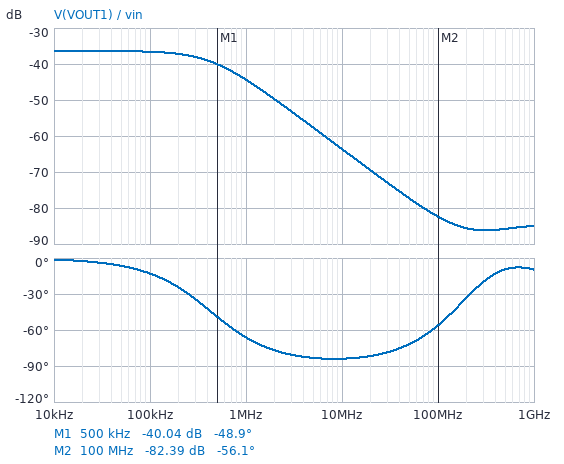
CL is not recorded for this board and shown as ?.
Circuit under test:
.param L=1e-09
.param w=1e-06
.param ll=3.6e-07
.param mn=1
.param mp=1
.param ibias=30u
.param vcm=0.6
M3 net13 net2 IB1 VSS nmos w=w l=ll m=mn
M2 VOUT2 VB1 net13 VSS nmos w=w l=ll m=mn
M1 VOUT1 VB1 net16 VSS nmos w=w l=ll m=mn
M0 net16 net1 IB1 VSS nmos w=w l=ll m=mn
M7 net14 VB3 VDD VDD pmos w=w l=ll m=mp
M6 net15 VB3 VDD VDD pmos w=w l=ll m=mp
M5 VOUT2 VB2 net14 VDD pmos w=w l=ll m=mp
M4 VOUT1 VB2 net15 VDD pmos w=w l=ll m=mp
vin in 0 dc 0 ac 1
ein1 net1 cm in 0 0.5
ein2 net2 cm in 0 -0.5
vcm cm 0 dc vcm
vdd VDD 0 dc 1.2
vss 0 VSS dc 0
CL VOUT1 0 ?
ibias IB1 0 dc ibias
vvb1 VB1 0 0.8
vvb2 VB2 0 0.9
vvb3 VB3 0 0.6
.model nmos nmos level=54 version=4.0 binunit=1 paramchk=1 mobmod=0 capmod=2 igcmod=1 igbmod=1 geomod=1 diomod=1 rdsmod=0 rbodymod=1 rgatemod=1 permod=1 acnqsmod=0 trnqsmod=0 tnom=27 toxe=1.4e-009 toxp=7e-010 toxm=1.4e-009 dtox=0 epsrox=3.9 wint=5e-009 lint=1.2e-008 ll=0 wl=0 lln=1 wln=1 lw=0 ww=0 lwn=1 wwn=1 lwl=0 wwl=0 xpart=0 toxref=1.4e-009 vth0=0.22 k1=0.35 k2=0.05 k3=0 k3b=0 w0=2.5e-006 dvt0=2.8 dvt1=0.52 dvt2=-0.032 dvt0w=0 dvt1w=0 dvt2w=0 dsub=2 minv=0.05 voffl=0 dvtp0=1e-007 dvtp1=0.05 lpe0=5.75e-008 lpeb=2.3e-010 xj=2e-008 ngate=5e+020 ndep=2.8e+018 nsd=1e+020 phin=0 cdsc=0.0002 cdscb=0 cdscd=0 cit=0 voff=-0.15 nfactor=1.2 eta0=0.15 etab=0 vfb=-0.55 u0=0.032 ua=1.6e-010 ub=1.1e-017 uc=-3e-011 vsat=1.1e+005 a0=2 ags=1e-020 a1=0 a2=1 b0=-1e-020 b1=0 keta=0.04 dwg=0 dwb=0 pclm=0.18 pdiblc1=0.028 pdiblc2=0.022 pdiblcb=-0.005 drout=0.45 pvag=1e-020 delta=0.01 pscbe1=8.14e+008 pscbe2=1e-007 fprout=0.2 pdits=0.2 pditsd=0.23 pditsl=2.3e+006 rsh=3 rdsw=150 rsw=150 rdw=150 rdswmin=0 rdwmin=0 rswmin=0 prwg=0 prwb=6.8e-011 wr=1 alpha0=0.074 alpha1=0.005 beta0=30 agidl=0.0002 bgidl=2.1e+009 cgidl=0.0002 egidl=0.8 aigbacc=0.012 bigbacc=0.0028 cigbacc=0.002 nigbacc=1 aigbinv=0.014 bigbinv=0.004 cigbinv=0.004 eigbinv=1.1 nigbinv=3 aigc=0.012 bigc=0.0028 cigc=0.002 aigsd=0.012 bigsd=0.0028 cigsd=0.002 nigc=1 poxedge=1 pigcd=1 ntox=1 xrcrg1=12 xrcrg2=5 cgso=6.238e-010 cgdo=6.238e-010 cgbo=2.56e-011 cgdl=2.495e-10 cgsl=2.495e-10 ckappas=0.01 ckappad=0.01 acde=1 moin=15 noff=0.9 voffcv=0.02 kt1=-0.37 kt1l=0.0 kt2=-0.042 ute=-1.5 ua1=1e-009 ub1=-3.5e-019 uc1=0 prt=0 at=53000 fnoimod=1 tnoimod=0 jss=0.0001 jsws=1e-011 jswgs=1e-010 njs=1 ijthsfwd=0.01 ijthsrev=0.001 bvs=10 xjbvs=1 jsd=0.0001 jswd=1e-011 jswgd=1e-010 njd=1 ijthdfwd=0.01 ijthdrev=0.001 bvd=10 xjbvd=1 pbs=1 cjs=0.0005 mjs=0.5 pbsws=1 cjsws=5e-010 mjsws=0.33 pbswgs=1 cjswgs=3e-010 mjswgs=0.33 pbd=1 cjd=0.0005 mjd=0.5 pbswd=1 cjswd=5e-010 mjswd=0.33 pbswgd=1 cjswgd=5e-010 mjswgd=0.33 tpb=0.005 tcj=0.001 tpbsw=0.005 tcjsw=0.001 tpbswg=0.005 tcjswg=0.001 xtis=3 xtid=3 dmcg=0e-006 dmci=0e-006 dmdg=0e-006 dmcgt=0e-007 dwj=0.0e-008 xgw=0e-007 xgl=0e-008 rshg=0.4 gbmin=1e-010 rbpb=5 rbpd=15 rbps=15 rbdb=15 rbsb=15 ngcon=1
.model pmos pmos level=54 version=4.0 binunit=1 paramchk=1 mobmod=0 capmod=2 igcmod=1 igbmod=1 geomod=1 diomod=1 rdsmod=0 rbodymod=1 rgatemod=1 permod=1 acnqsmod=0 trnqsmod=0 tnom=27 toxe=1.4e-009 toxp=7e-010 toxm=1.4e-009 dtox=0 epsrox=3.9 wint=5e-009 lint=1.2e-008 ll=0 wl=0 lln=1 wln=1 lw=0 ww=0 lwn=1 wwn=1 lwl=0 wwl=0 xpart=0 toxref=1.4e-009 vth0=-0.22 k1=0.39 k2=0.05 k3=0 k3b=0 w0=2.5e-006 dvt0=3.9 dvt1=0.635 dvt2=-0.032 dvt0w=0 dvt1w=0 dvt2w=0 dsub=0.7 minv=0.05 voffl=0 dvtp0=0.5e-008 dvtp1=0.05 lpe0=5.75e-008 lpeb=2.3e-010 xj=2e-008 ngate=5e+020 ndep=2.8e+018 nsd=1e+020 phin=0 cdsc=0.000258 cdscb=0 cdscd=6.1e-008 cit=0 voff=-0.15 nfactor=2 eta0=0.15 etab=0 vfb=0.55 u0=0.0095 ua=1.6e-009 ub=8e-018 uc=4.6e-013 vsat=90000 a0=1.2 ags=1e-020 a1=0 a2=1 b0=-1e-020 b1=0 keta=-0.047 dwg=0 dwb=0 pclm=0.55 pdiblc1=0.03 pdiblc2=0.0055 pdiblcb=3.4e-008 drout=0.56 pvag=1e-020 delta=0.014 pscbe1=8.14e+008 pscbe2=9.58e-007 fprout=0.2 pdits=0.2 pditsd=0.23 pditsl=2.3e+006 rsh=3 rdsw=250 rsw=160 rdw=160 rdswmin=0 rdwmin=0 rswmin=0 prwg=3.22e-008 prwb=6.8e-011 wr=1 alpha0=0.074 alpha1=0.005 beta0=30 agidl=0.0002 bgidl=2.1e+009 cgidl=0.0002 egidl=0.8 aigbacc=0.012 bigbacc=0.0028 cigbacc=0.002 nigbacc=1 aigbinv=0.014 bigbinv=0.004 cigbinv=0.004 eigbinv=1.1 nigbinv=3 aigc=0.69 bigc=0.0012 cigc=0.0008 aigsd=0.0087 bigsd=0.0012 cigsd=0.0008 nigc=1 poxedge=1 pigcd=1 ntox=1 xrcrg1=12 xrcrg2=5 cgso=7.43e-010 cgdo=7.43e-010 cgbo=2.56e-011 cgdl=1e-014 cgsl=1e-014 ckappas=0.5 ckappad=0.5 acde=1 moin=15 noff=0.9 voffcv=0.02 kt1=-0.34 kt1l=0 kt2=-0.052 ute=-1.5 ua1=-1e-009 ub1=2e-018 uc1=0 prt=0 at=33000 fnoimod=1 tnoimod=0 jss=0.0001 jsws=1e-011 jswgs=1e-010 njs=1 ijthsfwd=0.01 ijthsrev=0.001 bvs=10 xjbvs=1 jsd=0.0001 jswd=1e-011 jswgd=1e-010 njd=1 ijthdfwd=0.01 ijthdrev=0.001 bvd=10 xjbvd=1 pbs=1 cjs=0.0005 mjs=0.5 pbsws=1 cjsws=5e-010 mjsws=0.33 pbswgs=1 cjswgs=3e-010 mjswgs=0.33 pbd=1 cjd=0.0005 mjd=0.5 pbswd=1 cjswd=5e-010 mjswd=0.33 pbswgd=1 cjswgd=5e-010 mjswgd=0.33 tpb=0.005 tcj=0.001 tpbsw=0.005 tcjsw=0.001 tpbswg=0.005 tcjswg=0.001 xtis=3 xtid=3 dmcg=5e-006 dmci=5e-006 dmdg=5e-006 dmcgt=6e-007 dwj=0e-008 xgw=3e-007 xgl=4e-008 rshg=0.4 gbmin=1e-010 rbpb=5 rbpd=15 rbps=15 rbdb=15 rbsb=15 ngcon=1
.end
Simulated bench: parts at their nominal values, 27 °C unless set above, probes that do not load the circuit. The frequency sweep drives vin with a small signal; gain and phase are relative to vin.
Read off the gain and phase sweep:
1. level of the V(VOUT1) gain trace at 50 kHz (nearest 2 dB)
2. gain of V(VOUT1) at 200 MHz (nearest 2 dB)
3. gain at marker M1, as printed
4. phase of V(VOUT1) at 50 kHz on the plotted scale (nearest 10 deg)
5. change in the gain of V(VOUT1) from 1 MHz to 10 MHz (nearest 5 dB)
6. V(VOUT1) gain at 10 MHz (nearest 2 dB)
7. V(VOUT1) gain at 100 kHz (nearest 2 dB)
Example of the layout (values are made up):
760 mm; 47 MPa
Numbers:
-36 dB; -86 dB; -40.04 dB; -10 deg; -20 dB; -64 dB; -36 dB
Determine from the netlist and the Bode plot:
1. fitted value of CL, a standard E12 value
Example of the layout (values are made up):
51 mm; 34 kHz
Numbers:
33 pF
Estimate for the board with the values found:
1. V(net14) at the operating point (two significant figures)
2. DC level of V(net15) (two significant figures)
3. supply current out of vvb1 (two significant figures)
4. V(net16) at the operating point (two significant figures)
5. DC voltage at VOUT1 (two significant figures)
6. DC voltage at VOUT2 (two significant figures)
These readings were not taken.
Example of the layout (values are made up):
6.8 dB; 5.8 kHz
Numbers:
1.2 V; 1.2 V; 19 µA; -320 mV; -300 mV; -300 mV
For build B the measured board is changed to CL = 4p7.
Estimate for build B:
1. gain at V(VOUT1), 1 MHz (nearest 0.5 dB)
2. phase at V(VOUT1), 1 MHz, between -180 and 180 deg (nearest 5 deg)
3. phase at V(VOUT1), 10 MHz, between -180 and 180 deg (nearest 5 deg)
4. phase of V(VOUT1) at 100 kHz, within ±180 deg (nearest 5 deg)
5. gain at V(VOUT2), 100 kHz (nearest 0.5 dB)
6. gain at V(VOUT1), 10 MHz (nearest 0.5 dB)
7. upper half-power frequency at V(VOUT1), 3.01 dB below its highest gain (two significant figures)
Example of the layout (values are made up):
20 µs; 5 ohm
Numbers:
-37.0 dB; -20 deg; -70 deg; 0 deg; -36.5 dB; -47.0 dB; 3.0 MHz
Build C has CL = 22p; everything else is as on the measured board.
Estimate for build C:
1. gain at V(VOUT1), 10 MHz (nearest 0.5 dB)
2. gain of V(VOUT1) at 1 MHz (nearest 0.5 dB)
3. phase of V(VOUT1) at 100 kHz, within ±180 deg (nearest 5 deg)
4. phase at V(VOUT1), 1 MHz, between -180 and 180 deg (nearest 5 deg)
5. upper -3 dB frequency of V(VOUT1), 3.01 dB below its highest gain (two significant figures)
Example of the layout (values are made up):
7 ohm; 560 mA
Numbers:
-60.0 dB; -41.5 dB; -10 deg; -55 deg; 650 kHz
